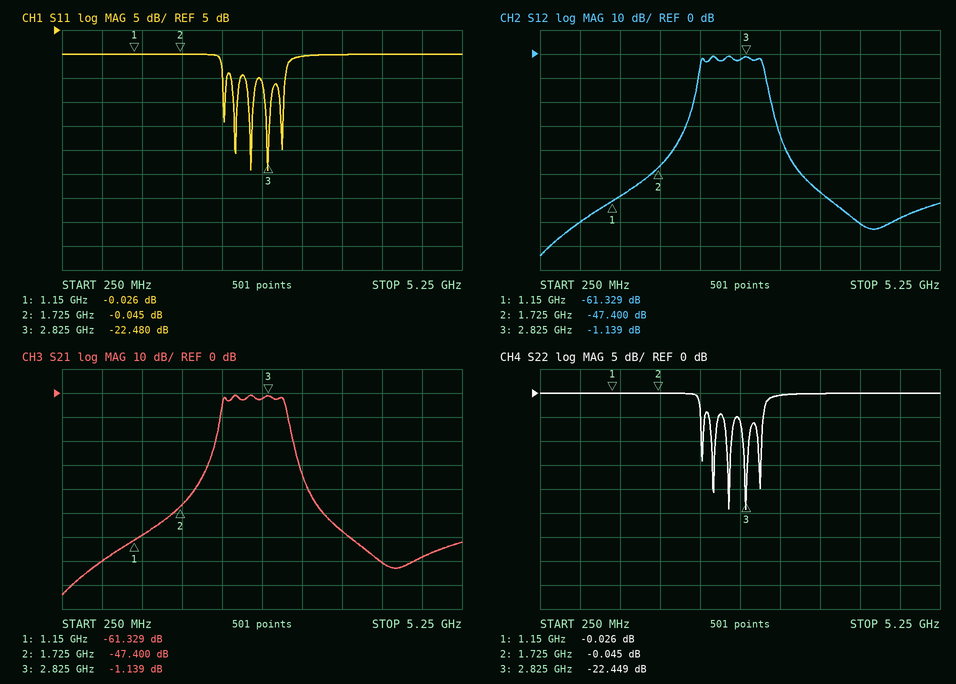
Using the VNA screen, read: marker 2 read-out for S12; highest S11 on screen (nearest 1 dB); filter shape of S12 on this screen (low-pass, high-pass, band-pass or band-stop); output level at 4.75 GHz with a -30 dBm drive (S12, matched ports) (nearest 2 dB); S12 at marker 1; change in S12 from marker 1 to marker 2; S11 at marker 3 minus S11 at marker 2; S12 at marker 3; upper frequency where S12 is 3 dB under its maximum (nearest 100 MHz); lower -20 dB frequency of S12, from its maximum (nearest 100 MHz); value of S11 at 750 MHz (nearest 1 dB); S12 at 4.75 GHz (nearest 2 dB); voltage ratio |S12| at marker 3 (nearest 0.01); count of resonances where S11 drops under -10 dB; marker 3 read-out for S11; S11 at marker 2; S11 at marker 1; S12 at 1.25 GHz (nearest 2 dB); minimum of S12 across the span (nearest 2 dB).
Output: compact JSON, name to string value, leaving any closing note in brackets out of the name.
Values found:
{"marker 2 read-out for S12": "-47.400 dB", "highest S11 on screen": "0 dB", "filter shape of S12 on this screen": "band-pass", "output level at 4.75 GHz with a -30 dBm drive (S12, matched ports)": "-98 dBm", "S12 at marker 1": "-61.329 dB", "change in S12 from marker 1 to marker 2": "13.929 dB", "S11 at marker 3 minus S11 at marker 2": "-22.435 dB", "S12 at marker 3": "-1.139 dB", "upper frequency where S12 is 3 dB under its maximum": "3.0 GHz", "lower -20 dB frequency of S12, from its maximum": "2.2 GHz", "value of S11 at 750 MHz": "0 dB", "S12 at 4.75 GHz": "-68 dB", "voltage ratio |S12| at marker 3": "0.88", "count of resonances where S11 drops under -10 dB": "5", "marker 3 read-out for S11": "-22.480 dB", "S11 at marker 2": "-0.045 dB", "S11 at marker 1": "-0.026 dB", "S12 at 1.25 GHz": "-60 dB", "minimum of S12 across the span": "-84 dB"}
